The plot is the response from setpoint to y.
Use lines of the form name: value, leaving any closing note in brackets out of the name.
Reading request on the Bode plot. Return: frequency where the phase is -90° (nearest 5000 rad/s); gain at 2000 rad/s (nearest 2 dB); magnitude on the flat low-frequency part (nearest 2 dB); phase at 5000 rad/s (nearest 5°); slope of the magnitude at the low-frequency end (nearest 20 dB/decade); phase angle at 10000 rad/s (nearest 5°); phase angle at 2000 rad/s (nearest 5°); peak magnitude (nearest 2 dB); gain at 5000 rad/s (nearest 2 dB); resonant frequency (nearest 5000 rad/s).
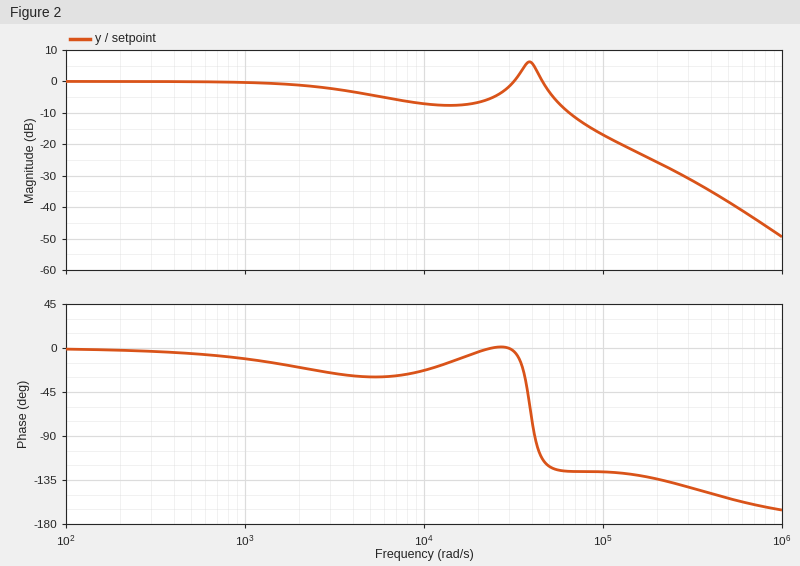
frequency where the phase is -90°: 40000 rad/s
gain at 2000 rad/s: -2 dB
magnitude on the flat low-frequency part: 0 dB
phase at 5000 rad/s: -30°
slope of the magnitude at the low-frequency end: 0 dB/decade
phase angle at 10000 rad/s: -25°
phase angle at 2000 rad/s: -20°
peak magnitude: 6 dB
gain at 5000 rad/s: -4 dB
resonant frequency: 40000 rad/s
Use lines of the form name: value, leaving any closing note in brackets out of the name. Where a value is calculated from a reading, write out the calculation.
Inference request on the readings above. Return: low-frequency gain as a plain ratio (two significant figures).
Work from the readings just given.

low-frequency gain as a plain ratio: 10^(0 / 20) = 1.0
